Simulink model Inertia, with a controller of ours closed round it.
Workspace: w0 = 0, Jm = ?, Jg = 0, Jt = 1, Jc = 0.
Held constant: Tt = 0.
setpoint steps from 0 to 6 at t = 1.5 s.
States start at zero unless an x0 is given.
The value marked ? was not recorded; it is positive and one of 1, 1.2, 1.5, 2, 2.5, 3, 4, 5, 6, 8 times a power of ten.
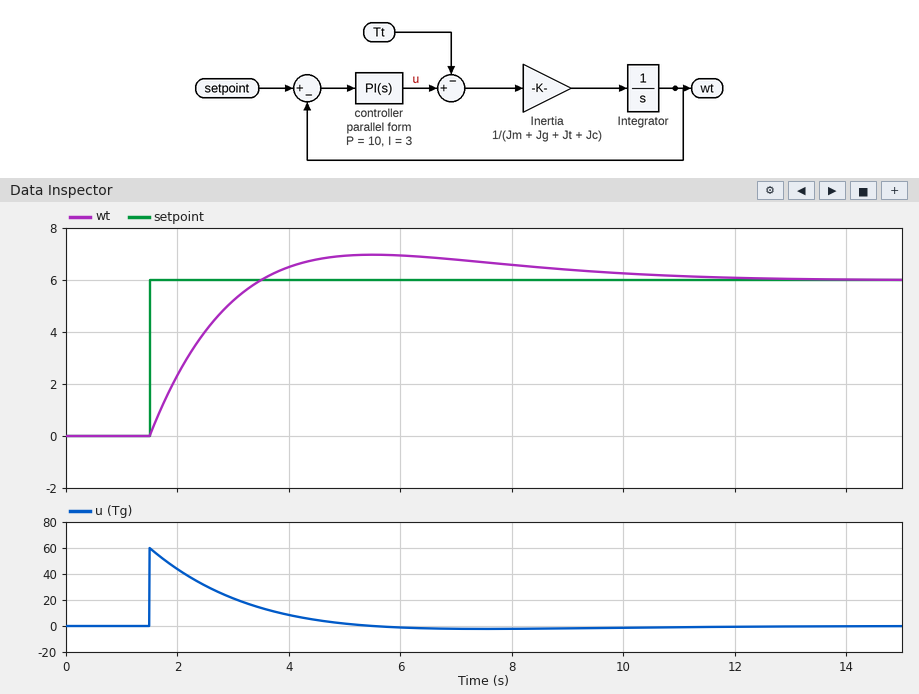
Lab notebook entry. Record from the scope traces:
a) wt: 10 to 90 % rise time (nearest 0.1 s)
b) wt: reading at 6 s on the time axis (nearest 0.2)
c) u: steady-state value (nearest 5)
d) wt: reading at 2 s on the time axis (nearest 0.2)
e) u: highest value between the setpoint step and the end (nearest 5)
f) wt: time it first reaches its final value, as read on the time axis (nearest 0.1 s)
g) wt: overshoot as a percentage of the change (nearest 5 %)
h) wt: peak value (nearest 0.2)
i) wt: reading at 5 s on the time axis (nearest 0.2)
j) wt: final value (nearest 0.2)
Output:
1.5 s
7.0
0
2.4
60
3.5 s
15 %
7.0
7.0
6.0
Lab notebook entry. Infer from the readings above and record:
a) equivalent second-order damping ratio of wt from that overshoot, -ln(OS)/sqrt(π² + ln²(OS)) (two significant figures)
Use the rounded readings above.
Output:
0.52
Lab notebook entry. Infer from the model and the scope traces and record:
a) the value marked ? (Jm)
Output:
10
